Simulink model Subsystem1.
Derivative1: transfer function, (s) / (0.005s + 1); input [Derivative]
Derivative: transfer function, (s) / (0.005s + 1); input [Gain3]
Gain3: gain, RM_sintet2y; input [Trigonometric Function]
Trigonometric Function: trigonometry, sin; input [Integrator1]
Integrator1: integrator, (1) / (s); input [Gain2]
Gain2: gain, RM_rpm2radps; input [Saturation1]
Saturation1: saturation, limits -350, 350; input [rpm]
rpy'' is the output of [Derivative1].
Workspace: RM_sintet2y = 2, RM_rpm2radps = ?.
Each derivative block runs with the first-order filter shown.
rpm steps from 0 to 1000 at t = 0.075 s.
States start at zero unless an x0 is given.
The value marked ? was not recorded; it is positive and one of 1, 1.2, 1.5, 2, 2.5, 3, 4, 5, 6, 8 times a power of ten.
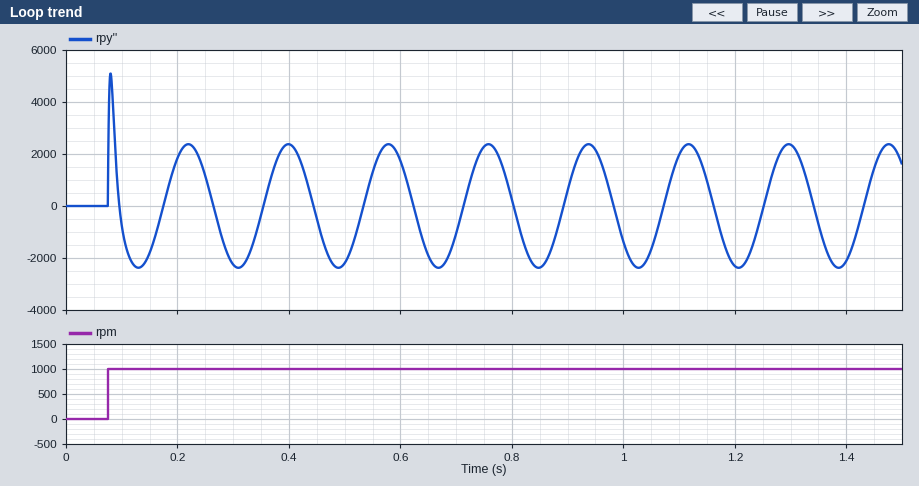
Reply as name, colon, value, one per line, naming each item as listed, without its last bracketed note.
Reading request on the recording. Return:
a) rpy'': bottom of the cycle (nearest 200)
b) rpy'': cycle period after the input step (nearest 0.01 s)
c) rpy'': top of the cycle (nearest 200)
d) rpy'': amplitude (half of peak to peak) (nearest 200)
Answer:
rpy'': bottom of the cycle: -2400
rpy'': cycle period after the input step: 0.18 s
rpy'': top of the cycle: 2400
rpy'': amplitude (half of peak to peak): 2400
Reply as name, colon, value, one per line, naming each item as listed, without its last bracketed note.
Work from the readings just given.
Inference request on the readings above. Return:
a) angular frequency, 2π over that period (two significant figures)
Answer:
angular frequency, 2π over that period: 35 rad/s
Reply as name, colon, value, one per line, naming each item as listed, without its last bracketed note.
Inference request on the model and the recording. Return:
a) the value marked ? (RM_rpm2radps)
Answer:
the value marked ?: 0.1
